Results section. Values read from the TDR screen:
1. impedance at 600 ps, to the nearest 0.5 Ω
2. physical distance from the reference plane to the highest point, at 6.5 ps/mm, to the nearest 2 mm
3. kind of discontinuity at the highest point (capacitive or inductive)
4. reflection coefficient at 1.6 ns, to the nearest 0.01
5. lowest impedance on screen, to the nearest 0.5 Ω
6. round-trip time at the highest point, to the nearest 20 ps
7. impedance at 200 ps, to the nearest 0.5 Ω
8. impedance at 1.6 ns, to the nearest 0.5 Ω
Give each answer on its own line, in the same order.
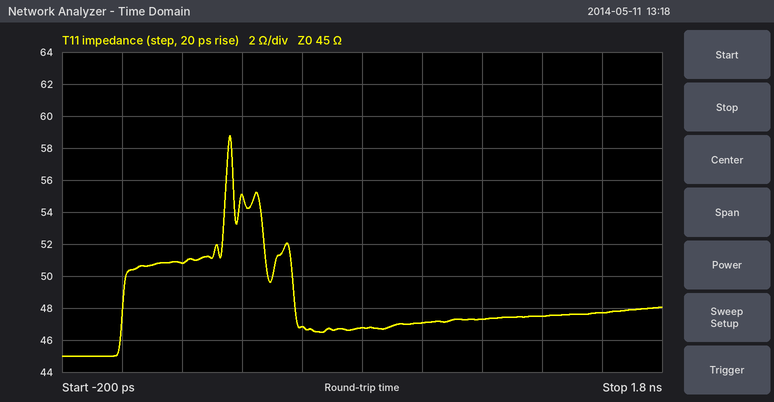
47.0 Ω
28 mm
inductive
+0.03
45.0 Ω
360 ps
51.0 Ω
47.5 Ω
